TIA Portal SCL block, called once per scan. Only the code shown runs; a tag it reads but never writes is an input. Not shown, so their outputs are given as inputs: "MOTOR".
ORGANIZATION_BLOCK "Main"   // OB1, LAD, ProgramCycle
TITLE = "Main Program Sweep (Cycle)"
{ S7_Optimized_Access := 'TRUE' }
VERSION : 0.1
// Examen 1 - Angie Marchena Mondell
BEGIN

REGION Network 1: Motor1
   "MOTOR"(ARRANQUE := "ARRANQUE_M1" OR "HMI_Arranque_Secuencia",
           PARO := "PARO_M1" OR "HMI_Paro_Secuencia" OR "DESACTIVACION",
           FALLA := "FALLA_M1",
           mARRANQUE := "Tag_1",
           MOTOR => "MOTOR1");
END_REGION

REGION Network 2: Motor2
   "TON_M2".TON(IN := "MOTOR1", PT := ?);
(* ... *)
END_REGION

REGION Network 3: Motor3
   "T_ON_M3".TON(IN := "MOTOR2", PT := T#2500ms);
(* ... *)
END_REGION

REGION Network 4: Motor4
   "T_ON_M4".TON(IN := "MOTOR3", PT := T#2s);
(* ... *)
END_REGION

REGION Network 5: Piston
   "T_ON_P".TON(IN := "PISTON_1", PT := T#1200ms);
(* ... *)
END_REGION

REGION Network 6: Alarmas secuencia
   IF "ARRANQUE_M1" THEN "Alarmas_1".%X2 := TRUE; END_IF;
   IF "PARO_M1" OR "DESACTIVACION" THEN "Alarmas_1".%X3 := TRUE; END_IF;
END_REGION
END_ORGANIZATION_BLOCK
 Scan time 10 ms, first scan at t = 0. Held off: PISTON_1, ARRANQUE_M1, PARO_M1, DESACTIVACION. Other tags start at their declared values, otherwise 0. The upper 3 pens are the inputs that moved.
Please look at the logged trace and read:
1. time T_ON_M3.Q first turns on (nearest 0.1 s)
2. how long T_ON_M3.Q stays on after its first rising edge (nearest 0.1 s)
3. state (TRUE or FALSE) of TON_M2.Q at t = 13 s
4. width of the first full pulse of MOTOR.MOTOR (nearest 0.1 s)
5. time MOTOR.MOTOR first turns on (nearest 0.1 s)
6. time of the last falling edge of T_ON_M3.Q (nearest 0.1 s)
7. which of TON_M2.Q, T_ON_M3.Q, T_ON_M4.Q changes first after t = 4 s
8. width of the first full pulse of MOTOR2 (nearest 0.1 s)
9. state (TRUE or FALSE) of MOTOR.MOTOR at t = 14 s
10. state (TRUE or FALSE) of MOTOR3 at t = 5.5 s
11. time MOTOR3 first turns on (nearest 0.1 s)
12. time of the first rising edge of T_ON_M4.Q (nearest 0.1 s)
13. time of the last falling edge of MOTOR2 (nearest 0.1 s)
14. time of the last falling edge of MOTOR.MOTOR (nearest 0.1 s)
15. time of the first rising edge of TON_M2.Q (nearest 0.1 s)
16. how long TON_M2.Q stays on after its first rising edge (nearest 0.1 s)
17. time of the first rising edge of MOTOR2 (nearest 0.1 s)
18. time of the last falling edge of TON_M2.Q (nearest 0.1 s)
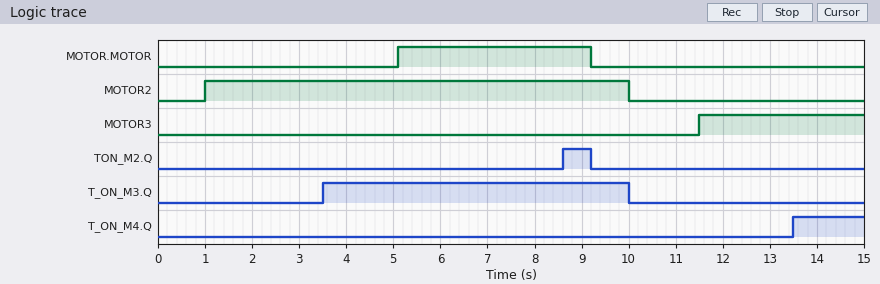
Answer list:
3.5 s
6.5 s
FALSE
4.1 s
5.1 s
10.0 s
TON_M2.Q
9.0 s
FALSE
FALSE
11.5 s
13.5 s
10.0 s
9.2 s
8.6 s
0.6 s
1.0 s
9.2 s
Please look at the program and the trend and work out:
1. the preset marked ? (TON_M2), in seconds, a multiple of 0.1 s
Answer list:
3.5 s
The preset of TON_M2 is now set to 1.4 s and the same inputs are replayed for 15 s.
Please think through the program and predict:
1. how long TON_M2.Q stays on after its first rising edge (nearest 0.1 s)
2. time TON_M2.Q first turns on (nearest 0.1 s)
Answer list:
2.7 s
6.5 s
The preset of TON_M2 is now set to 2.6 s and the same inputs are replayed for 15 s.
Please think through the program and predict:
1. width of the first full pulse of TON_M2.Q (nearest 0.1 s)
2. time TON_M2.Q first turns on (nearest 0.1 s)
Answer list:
1.5 s
7.7 s
